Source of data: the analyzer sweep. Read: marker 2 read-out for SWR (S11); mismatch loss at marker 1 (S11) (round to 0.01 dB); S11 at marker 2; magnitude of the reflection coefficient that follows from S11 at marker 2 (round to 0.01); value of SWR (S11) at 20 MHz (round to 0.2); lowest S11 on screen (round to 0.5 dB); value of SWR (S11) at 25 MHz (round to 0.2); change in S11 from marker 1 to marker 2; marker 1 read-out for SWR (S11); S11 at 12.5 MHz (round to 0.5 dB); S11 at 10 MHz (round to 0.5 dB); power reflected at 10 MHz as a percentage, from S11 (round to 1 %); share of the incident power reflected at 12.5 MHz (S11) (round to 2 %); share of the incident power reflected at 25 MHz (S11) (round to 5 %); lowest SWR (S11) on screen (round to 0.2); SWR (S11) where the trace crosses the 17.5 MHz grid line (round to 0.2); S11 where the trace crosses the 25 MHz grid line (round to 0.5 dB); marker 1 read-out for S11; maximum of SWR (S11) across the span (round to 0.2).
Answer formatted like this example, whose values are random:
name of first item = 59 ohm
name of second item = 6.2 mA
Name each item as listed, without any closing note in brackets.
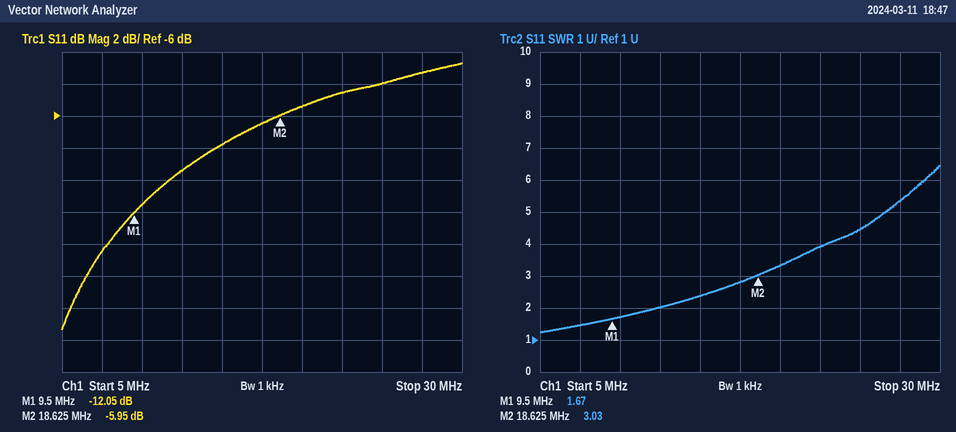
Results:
marker 2 read-out for SWR = 3.03
mismatch loss at marker 1 (S11) = 0.28 dB
S11 at marker 2 = -5.95 dB
magnitude of the reflection coefficient that follows from S11 at marker 2 = 0.50
value of SWR (S11) at 20 MHz = 3.4
lowest S11 on screen = -19.5 dB
value of SWR (S11) at 25 MHz = 4.4
change in S11 from marker 1 to marker 2 = 6.10 dB
marker 1 read-out for SWR = 1.67
S11 at 12.5 MHz = -9.5 dB
S11 at 10 MHz = -11.5 dB
power reflected at 10 MHz as a percentage, from S11 = 7 %
share of the incident power reflected at 12.5 MHz (S11) = 12 %
share of the incident power reflected at 25 MHz (S11) = 40 %
lowest SWR (S11) on screen = 1.2
SWR (S11) where the trace crosses the 17.5 MHz grid line = 2.8
S11 where the trace crosses the 25 MHz grid line = -4.0 dB
marker 1 read-out for S11 = -12.05 dB
maximum of SWR (S11) across the span = 6.4
